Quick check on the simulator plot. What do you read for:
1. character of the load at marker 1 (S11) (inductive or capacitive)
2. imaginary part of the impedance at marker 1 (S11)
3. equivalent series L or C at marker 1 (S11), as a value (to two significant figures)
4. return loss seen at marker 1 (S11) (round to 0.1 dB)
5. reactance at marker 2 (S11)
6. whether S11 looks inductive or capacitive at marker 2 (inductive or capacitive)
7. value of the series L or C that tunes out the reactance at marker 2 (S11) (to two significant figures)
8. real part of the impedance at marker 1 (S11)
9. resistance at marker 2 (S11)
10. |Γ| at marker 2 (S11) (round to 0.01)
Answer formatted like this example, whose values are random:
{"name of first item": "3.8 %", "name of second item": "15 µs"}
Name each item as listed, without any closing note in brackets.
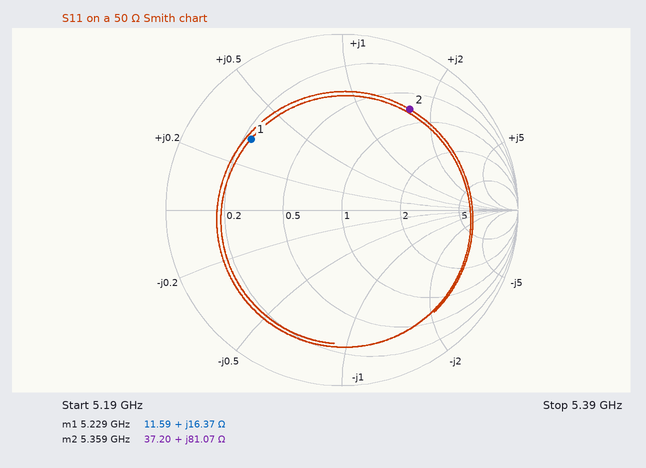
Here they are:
{"character of the load at marker 1 (S11)": "inductive", "imaginary part of the impedance at marker 1": "+16.37 Ω", "equivalent series L or C at marker 1 (S11), as a value": "500 pH", "return loss seen at marker 1 (S11)": "3.7 dB", "reactance at marker 2": "+81.07 Ω", "whether S11 looks inductive or capacitive at marker 2": "inductive", "value of the series L or C that tunes out the reactance at marker 2 (S11)": "370 fF", "real part of the impedance at marker 1": "11.59 Ω", "resistance at marker 2": "37.20 Ω", "|Γ| at marker 2 (S11)": "0.69"}
